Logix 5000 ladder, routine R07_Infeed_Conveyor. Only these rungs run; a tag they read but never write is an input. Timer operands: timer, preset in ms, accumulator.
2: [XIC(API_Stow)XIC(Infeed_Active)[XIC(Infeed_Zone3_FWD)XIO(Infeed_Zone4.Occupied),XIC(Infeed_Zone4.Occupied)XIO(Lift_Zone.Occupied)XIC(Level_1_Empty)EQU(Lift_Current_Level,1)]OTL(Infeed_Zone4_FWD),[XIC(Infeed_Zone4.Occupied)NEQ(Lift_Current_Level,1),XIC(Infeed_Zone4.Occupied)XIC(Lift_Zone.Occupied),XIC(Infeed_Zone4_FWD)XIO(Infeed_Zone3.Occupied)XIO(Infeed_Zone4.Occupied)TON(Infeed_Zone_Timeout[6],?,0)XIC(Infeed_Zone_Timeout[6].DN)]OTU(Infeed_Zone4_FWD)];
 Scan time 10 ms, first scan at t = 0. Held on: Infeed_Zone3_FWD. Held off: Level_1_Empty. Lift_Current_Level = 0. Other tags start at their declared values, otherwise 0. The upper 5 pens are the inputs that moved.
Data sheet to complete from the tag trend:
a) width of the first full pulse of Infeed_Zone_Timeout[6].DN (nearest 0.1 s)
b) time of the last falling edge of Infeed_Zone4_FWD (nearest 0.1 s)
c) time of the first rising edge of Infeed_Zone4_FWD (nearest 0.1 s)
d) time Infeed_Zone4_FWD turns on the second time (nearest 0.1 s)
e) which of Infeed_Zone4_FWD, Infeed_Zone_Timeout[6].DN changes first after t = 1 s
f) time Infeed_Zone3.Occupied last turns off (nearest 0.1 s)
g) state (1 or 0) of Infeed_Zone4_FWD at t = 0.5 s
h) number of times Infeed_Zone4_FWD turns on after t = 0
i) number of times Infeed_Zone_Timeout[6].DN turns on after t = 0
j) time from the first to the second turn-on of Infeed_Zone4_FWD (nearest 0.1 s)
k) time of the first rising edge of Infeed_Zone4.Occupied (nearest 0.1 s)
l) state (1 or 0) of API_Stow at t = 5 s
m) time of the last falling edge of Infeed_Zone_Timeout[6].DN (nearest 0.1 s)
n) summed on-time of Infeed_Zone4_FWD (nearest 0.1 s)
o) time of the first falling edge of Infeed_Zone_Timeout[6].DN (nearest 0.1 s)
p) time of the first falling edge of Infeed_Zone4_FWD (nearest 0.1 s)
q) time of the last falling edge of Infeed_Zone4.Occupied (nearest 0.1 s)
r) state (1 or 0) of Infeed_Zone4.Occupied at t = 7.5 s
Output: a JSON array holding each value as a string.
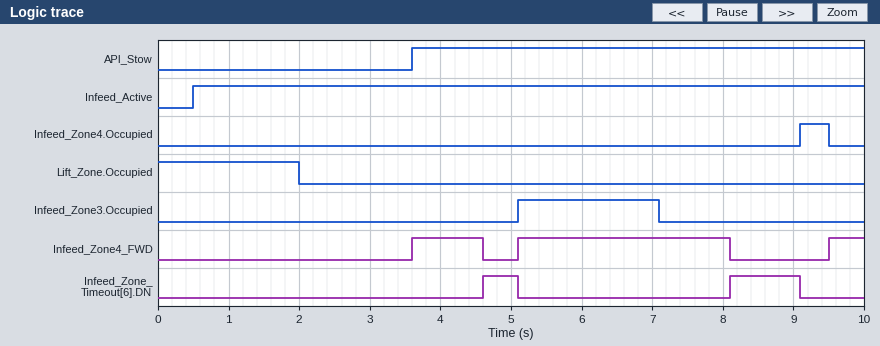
["0.5 s", "8.1 s", "3.6 s", "5.1 s", "Infeed_Zone4_FWD", "7.1 s", "0", "3", "2", "1.5 s", "9.1 s", "1", "9.1 s", "4.5 s", "5.1 s", "4.6 s", "9.5 s", "0"]
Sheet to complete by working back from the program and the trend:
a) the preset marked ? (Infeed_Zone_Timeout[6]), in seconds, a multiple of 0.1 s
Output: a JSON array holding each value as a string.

["1.0 s"]
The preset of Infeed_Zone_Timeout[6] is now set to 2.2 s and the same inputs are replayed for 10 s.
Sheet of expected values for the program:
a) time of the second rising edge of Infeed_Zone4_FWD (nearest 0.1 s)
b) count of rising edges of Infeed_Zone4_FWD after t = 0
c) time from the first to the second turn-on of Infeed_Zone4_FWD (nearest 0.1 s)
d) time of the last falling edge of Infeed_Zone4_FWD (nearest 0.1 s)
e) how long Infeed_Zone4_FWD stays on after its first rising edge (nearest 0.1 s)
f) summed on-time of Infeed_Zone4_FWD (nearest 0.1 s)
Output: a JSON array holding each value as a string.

["9.5 s", "2", "5.9 s", "9.1 s", "5.5 s", "6.0 s"]
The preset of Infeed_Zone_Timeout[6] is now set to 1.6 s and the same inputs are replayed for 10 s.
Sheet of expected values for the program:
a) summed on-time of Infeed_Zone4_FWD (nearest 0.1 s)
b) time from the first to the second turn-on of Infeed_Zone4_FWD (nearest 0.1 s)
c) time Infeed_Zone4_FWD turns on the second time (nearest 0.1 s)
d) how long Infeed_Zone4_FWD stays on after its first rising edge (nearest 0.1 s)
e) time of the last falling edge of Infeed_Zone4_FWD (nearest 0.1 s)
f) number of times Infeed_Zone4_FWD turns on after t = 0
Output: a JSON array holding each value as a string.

["5.6 s", "5.9 s", "9.5 s", "5.1 s", "8.7 s", "2"]
